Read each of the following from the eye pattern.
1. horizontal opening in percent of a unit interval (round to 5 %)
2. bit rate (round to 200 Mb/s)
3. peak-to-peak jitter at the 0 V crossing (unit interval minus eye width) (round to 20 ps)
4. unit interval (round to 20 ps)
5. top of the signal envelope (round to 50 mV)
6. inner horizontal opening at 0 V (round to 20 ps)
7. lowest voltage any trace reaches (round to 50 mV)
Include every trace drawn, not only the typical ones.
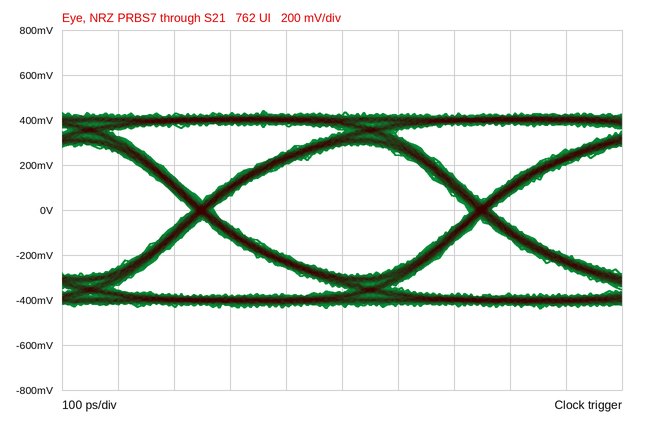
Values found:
90 %
2.0 Gb/s
40 ps
500 ps
450 mV
460 ps
-450 mV
